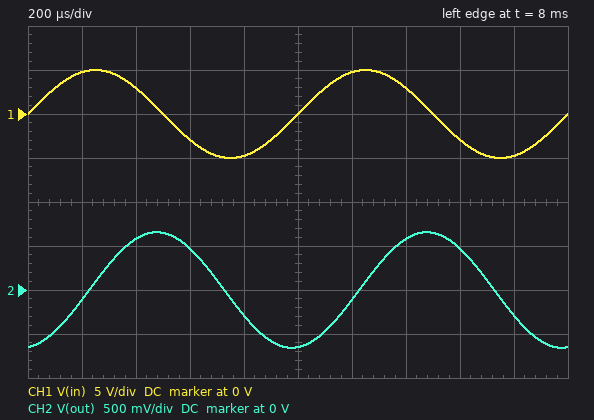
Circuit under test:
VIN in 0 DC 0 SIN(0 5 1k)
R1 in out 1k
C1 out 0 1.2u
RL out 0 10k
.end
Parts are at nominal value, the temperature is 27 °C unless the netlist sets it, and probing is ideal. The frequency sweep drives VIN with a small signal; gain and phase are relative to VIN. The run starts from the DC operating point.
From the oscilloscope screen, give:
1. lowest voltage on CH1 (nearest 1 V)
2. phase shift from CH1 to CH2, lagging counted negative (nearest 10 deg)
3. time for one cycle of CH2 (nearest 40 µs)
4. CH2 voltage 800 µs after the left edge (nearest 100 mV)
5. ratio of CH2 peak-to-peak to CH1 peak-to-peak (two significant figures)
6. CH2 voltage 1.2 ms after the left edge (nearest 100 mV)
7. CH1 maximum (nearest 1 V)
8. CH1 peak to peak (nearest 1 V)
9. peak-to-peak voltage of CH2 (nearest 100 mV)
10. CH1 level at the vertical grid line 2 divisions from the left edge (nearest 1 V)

-5 V
-80 deg
1.00 ms
-300 mV
0.13
-100 mV
5 V
10 V
1.3 V
3 V
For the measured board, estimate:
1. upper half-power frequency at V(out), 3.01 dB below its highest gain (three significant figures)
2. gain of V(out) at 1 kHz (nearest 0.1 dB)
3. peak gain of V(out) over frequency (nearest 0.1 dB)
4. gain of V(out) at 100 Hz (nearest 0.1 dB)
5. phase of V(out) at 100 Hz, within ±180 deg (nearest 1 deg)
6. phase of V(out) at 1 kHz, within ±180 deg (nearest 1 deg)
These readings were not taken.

146 Hz
-17.6 dB
-0.8 dB
-2.5 dB
-34 deg
-82 deg
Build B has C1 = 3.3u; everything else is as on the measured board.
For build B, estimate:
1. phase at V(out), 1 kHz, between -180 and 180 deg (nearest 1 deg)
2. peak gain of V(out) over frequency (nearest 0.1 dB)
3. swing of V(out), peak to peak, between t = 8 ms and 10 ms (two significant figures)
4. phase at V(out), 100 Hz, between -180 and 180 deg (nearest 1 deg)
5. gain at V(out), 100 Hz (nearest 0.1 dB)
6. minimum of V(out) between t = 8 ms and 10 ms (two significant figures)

-87 deg
-0.8 dB
490 mV
-62 deg
-7.4 dB
-230 mV
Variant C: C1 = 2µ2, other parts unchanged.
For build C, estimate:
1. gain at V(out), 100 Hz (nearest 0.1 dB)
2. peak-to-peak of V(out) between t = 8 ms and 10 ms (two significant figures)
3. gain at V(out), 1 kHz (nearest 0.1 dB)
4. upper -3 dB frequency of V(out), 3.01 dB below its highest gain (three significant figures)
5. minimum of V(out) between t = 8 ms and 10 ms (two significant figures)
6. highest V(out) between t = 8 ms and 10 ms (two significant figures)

-4.9 dB
720 mV
-22.8 dB
79.6 Hz
-360 mV
370 mV
